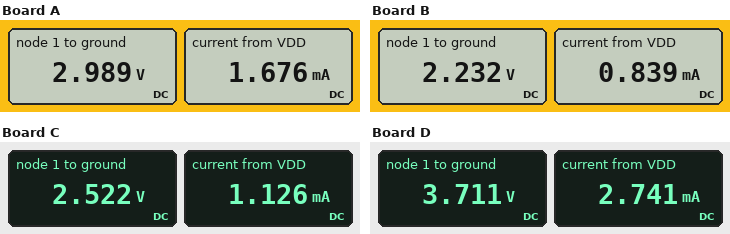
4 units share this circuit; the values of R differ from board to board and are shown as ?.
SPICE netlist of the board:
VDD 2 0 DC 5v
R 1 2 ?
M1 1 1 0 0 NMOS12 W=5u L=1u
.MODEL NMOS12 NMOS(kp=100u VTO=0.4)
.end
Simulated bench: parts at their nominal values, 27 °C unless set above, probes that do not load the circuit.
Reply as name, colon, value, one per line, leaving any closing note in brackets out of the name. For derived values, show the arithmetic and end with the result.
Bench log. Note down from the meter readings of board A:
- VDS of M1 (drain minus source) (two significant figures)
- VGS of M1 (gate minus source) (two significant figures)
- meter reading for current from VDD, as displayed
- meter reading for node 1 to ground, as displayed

VDS of M1 (drain minus source): 2.989 V = 3.0 V
VGS of M1 (gate minus source): 2.989 V = 3.0 V
meter reading for current from VDD, as displayed: 1.676 mA
meter reading for node 1 to ground, as displayed: 2.989 V
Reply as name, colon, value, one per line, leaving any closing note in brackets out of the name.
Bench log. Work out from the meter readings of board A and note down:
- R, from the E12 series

R, from the E12 series: 1.2 kΩ
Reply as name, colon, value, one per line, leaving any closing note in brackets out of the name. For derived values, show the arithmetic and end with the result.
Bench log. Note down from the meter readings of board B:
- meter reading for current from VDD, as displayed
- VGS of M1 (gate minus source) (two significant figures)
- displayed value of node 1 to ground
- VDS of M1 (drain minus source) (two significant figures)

meter reading for current from VDD, as displayed: 0.839 mA
VGS of M1 (gate minus source): 2.232 V = 2.2 V
displayed value of node 1 to ground: 2.232 V
VDS of M1 (drain minus source): 2.232 V = 2.2 V
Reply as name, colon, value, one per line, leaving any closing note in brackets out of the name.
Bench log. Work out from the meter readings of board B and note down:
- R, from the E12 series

R, from the E12 series: 3.3 kΩ
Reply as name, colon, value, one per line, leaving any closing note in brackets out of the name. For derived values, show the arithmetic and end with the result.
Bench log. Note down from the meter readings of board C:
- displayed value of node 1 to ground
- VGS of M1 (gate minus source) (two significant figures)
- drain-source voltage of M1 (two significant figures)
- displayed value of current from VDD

displayed value of node 1 to ground: 2.522 V
VGS of M1 (gate minus source): 2.522 V = 2.5 V
drain-source voltage of M1: 2.522 V = 2.5 V
displayed value of current from VDD: 1.126 mA
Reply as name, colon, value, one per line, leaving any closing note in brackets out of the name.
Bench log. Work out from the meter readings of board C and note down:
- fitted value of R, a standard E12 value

fitted value of R, a standard E12 value: 2.2 kΩ
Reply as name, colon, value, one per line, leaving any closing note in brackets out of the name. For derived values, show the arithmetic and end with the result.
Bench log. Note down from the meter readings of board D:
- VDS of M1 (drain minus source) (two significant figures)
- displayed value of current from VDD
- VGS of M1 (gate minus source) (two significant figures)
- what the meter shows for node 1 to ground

VDS of M1 (drain minus source): 3.711 V = 3.7 V
displayed value of current from VDD: 2.741 mA
VGS of M1 (gate minus source): 3.711 V = 3.7 V
what the meter shows for node 1 to ground: 3.711 V
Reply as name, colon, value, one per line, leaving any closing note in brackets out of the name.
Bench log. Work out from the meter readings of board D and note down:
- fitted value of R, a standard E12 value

fitted value of R, a standard E12 value: 470 Ω
